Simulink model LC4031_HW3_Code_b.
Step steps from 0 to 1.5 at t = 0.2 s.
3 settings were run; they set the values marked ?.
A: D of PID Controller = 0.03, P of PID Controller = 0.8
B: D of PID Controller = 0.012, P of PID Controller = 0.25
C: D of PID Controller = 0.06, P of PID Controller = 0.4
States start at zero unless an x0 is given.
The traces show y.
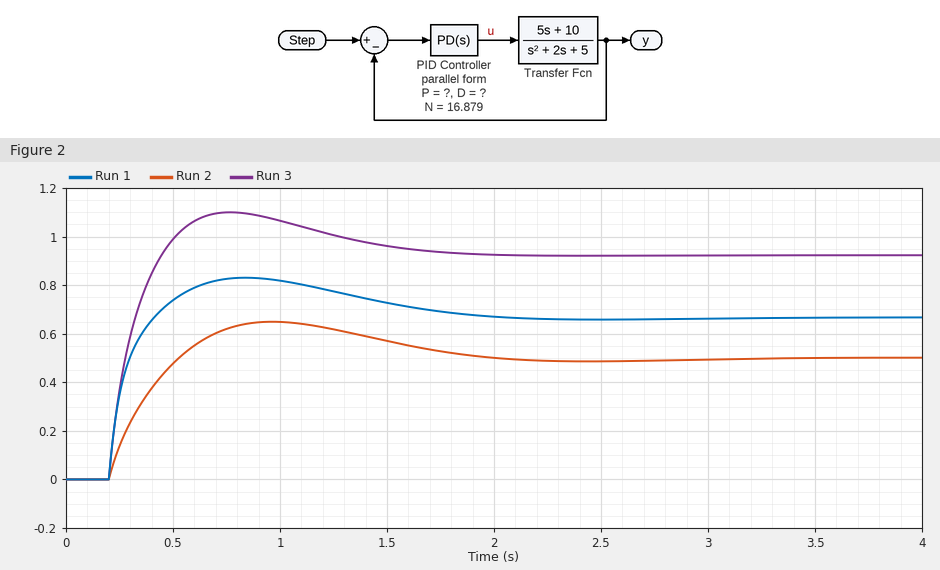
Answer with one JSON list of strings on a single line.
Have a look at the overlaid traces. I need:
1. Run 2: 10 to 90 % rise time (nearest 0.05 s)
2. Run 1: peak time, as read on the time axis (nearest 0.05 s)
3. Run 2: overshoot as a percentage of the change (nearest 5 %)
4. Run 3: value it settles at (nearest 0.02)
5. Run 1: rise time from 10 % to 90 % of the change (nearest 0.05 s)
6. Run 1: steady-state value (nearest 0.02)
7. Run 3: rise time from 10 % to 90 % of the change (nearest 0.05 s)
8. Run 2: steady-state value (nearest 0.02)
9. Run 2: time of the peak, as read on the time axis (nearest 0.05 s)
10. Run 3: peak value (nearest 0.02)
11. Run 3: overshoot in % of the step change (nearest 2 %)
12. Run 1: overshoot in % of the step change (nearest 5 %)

["0.25 s", "0.85 s", "30 %", "0.92", "0.15 s", "0.66", "0.20 s", "0.50", "0.95 s", "1.10", "20 %", "25 %"]
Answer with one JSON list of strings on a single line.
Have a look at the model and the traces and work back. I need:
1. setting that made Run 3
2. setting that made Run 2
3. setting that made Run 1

["A", "B", "C"]
